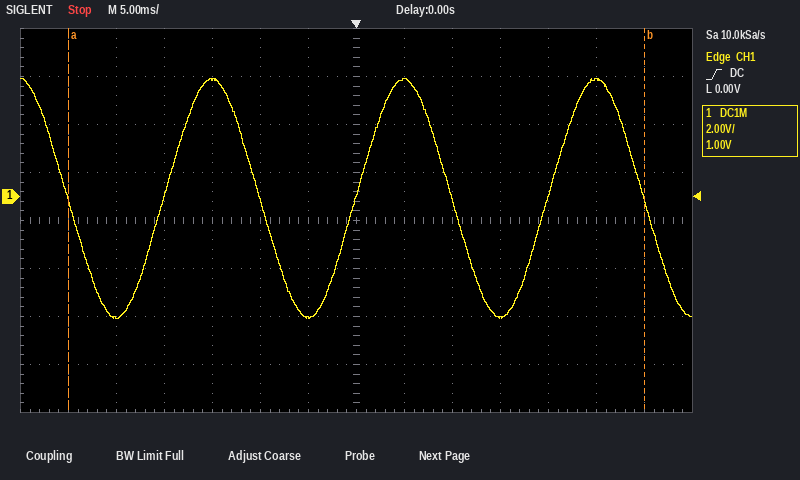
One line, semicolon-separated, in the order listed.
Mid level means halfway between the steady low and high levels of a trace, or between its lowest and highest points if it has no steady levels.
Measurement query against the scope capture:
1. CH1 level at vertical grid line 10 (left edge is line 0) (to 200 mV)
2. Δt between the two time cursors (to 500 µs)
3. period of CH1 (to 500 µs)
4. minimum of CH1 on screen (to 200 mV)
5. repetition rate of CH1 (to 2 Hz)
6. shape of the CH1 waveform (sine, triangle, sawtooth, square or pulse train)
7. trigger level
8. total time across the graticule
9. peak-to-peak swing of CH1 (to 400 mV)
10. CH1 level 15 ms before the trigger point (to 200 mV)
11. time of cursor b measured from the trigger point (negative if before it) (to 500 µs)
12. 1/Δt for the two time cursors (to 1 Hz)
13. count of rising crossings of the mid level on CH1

-5.0 V; 60.0 ms; 20.0 ms; -5.0 V; 50 Hz; sine; 0.00 V; 70 ms; 10.0 V; 4.8 V; +30.0 ms; 17 Hz; 3
